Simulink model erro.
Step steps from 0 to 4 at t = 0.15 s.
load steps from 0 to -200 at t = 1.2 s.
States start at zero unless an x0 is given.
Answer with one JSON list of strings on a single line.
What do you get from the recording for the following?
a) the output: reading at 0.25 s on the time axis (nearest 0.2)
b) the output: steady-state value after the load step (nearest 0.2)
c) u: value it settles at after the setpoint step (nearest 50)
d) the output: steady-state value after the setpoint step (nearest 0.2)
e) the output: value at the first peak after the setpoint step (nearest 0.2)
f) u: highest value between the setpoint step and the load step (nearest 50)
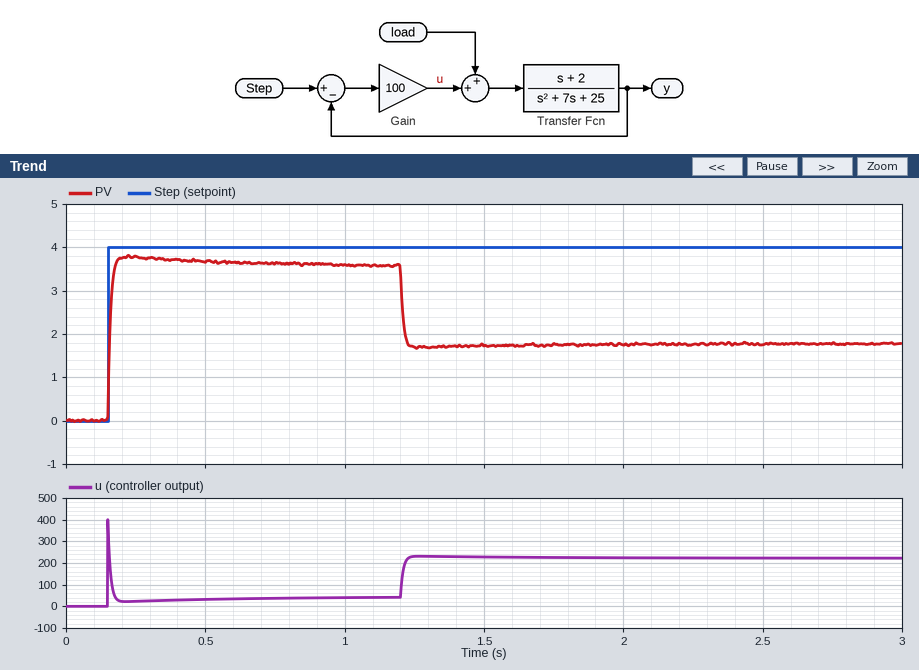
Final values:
["3.8", "1.8", "50", "3.6", "3.8", "400"]
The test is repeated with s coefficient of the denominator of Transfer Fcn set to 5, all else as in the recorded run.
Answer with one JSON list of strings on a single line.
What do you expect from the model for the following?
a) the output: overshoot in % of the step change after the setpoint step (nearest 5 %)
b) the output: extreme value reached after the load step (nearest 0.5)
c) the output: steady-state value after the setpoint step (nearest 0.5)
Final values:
["10 %", "1.5", "3.5"]
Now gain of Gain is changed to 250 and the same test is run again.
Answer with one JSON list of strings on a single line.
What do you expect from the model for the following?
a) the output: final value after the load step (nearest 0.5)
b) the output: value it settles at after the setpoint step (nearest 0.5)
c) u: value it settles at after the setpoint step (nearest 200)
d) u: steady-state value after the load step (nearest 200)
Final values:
["3.0", "4.0", "0", "200"]
